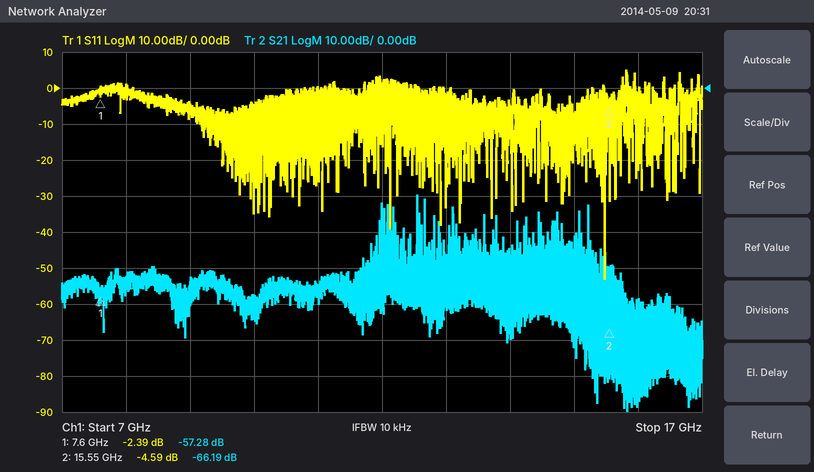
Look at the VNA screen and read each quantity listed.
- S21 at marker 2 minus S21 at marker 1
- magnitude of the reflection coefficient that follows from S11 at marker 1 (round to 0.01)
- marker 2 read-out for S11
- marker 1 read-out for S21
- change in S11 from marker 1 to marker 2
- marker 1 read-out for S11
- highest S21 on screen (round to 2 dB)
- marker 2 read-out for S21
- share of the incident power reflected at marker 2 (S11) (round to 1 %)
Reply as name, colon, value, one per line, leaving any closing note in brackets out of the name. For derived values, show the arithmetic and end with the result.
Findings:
S21 at marker 2 minus S21 at marker 1: -66.19 − (-57.28) = -8.91 dB
magnitude of the reflection coefficient that follows from S11 at marker 1: 10^(-2.39/20) ≈ 0.76
marker 2 read-out for S11: -4.59 dB
marker 1 read-out for S21: -57.28 dB
change in S11 from marker 1 to marker 2: -4.59 − (-2.39) = -2.20 dB
marker 1 read-out for S11: -2.39 dB
highest S21 on screen: -30 dB
marker 2 read-out for S21: -66.19 dB
share of the incident power reflected at marker 2 (S11): 10^(-4.59/10) ≈ 35 %
